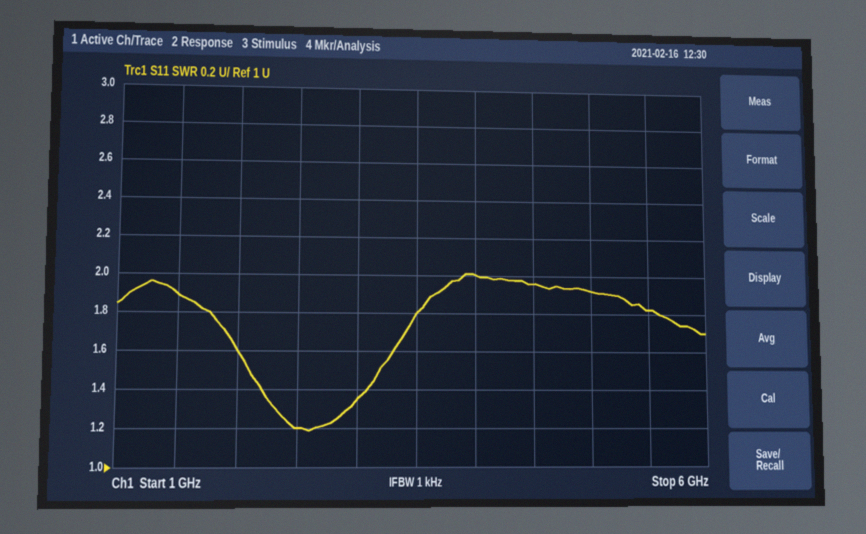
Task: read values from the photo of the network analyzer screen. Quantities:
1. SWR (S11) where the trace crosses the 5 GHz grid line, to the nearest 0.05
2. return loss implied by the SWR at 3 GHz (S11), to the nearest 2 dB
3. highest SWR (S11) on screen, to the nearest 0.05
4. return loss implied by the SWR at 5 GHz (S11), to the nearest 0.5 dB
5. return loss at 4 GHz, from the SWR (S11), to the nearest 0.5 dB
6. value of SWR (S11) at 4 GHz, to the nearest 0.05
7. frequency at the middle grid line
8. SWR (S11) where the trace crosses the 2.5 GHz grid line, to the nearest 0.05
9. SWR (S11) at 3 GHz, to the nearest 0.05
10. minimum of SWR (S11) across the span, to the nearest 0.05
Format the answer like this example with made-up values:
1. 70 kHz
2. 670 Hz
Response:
1. 1.90
2. 16 dB
3. 2.00
4. 10.0 dB
5. 9.5 dB
6. 2.00
7. 3.5 GHz
8. 1.20
9. 1.35
10. 1.20
